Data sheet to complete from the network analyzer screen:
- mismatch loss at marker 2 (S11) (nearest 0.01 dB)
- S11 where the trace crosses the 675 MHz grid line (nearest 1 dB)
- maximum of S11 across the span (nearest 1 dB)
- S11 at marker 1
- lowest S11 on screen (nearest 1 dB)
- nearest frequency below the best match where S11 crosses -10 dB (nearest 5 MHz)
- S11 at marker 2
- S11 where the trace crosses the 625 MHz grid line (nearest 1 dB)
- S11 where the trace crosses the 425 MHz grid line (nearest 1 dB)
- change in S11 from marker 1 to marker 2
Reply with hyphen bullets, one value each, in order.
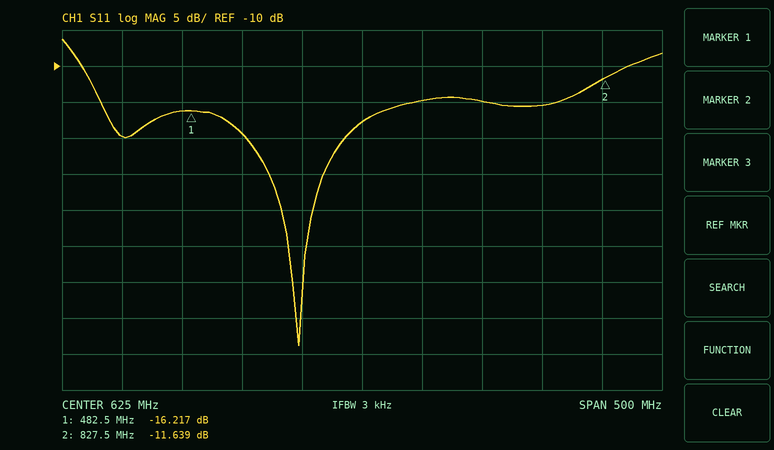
- 0.31 dB
- -15 dB
- -6 dB
- -16.217 dB
- -49 dB
- 390 MHz
- -11.639 dB
- -18 dB
- -20 dB
- 4.578 dB
